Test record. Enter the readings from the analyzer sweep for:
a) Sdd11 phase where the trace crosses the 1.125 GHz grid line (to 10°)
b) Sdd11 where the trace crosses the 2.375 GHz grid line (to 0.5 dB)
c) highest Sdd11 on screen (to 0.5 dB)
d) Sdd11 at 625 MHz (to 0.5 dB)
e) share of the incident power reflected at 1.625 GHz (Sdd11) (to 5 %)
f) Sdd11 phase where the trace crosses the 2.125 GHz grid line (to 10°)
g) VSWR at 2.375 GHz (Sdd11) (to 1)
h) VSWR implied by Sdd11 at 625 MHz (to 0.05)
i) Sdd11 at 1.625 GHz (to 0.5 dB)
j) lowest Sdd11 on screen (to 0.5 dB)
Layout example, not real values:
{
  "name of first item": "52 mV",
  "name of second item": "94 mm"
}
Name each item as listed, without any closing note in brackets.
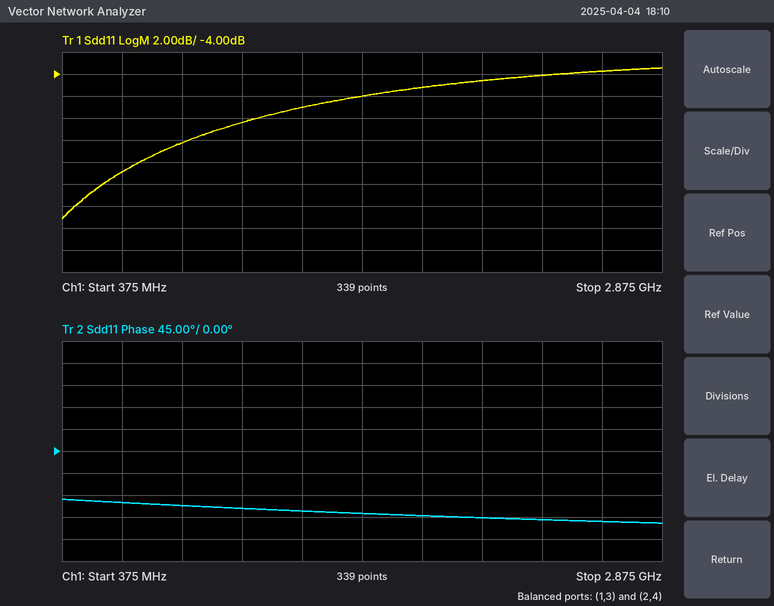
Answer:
{
  "Sdd11 phase where the trace crosses the 1.125 GHz grid line": "-120°",
  "Sdd11 where the trace crosses the 2.375 GHz grid line": "-4.0 dB",
  "highest Sdd11 on screen": "-3.5 dB",
  "Sdd11 at 625 MHz": "-13.0 dB",
  "share of the incident power reflected at 1.625 GHz (Sdd11)": "25 %",
  "Sdd11 phase where the trace crosses the 2.125 GHz grid line": "-140°",
  "VSWR at 2.375 GHz (Sdd11)": "4",
  "VSWR implied by Sdd11 at 625 MHz": "1.60",
  "Sdd11 at 1.625 GHz": "-6.0 dB",
  "lowest Sdd11 on screen": "-17.0 dB"
}
